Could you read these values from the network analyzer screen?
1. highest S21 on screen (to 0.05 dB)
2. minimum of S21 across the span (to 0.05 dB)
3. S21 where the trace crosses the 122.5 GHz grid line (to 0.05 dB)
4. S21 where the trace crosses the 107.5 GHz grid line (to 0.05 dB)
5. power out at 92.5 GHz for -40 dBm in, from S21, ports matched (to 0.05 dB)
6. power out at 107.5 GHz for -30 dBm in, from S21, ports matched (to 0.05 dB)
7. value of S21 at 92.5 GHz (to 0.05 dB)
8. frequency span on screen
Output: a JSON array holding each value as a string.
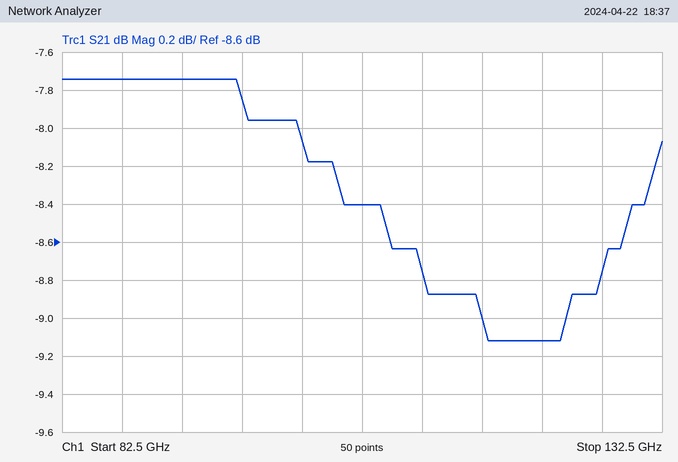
["-7.75 dB", "-9.10 dB", "-9.10 dB", "-8.40 dB", "-47.75 dBm", "-38.40 dBm", "-7.75 dB", "50 GHz"]
